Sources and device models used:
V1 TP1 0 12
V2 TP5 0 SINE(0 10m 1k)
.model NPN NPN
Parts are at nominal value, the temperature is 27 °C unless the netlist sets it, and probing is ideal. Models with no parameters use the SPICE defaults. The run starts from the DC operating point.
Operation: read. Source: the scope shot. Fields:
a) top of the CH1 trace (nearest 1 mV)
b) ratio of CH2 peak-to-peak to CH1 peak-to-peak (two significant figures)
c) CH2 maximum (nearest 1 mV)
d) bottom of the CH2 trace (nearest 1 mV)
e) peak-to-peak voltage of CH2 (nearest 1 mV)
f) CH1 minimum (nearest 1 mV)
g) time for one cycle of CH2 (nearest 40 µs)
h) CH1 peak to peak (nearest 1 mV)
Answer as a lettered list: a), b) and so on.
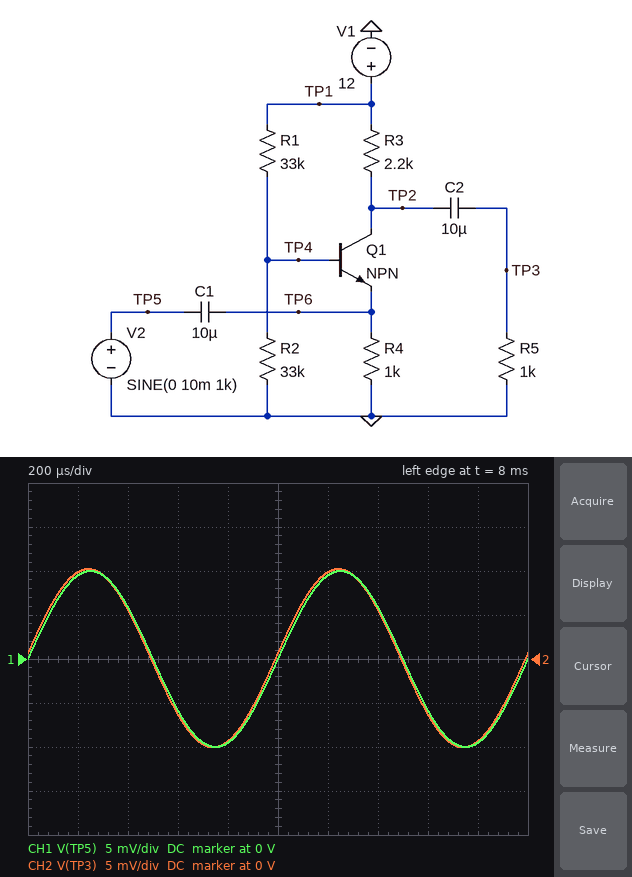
a) 10 mV
b) 1.0
c) 10 mV
d) -10 mV
e) 20 mV
f) -10 mV
g) 1.00 ms
h) 20 mV
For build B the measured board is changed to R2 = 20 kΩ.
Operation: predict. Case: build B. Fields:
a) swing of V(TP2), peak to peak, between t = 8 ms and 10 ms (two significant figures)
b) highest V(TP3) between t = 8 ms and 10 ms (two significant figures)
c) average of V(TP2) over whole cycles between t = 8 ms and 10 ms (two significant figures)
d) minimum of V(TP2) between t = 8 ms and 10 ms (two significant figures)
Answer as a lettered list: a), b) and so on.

a) 100 mV
b) 51 mV
c) 4.8 V
d) 4.7 V
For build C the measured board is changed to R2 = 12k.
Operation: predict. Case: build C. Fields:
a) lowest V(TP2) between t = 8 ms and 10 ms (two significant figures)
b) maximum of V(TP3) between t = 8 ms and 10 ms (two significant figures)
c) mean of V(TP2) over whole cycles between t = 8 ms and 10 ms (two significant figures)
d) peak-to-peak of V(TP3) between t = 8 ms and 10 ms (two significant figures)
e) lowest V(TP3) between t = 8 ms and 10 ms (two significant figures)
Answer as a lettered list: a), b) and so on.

a) 7.1 V
b) 68 mV
c) 7.2 V
d) 140 mV
e) -68 mV
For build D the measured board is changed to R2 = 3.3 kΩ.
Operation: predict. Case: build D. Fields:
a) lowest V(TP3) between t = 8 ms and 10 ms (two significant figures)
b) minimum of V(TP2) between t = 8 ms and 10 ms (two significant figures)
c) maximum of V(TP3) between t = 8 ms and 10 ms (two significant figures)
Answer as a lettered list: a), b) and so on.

a) -66 mV
b) 11 V
c) 59 mV
